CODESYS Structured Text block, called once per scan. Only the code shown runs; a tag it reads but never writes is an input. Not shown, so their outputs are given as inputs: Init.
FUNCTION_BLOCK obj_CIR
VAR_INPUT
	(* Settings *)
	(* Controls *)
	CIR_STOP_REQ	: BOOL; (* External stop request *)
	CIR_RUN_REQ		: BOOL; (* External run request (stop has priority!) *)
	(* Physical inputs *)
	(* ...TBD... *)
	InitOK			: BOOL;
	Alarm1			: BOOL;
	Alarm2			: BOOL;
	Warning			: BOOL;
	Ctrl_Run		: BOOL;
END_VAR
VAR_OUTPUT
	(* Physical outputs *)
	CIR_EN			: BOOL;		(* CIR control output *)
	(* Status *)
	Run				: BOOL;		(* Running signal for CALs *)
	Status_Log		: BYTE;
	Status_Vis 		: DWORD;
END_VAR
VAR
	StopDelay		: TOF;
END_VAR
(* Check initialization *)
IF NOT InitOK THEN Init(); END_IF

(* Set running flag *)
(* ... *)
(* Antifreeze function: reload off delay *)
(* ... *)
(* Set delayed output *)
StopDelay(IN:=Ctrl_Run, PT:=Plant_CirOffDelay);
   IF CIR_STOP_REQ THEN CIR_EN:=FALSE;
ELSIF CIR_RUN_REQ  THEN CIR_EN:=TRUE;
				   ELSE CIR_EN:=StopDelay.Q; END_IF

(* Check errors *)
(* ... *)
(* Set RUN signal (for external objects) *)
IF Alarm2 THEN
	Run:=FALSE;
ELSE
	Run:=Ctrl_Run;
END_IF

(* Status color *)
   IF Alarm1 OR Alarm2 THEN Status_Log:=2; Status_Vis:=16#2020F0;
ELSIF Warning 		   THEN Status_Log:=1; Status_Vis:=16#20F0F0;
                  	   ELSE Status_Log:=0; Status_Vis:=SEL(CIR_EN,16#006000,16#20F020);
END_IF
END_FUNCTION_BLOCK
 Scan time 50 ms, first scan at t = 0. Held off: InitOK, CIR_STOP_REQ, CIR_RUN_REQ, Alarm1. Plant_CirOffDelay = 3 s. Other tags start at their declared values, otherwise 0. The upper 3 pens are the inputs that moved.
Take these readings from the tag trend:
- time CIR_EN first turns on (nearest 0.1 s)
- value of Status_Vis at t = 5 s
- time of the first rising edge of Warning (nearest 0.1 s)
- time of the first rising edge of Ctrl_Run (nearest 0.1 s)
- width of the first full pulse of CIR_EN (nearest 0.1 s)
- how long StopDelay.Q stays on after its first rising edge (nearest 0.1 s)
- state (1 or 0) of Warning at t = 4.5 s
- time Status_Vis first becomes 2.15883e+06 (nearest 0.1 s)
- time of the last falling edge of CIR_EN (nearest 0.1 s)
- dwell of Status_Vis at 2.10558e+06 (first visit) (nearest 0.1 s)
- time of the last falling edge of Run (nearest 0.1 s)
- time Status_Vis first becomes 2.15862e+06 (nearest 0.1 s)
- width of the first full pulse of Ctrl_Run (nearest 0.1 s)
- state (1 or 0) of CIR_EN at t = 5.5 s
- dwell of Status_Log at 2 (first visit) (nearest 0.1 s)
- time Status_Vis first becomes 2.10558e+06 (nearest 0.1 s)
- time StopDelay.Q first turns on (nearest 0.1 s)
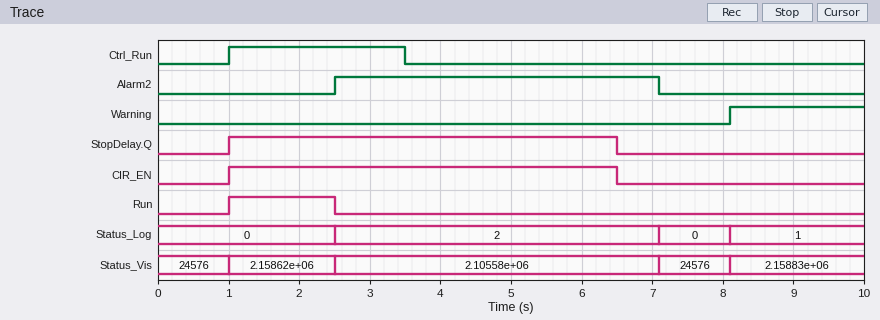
1.0 s
2.10558e+06
8.1 s
1.0 s
5.5 s
5.5 s
0
8.1 s
6.5 s
4.6 s
2.5 s
1.0 s
2.5 s
1
4.6 s
2.5 s
1.0 s
